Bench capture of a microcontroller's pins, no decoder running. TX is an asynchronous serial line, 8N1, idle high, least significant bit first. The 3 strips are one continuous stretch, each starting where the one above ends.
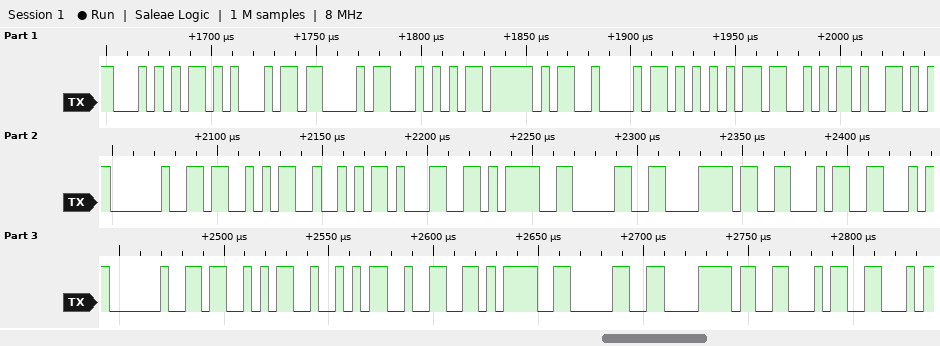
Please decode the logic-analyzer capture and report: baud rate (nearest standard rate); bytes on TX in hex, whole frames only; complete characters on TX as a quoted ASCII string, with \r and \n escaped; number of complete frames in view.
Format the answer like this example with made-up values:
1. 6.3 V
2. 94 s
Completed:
1. 250000 baud
2. 54 45 43 54 5F 42 55 53 59 20 53 52 31 3D 30 78 46 46 20 53 52 32 3D 30 78 46 46
3. "TECT_BUSY SR1=0xFF SR2=0xFF"
4. 27
